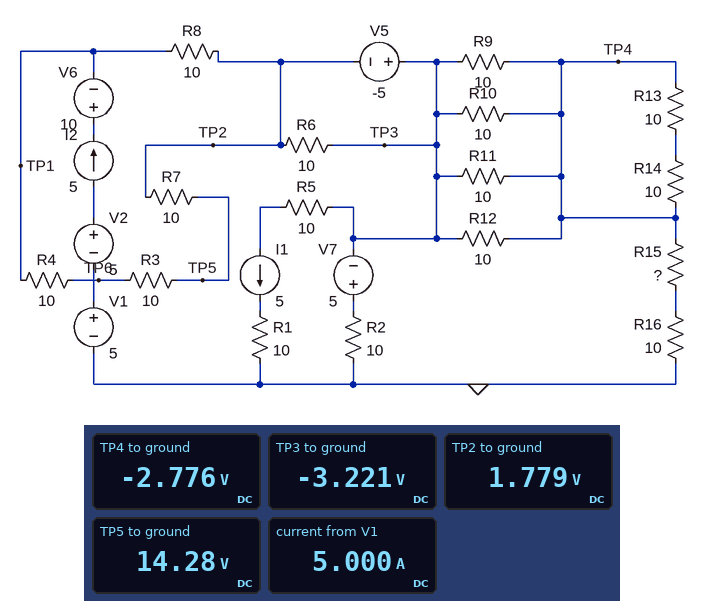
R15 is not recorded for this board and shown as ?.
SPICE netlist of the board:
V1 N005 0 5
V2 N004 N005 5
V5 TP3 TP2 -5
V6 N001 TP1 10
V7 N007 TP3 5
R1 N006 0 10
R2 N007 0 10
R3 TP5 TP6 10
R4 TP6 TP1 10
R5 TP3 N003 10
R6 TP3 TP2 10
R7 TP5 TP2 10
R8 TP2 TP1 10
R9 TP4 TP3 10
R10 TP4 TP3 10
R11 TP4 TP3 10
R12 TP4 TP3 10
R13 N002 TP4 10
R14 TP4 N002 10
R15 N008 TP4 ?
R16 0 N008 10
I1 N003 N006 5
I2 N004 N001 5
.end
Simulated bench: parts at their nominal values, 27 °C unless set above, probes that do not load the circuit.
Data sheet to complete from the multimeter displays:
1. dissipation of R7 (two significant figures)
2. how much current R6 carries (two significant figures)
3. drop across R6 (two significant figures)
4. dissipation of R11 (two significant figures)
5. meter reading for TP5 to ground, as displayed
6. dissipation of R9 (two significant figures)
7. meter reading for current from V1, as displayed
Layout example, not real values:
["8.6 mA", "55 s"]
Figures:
["16 W", "500 mA", "5.0 V", "20 mW", "14.28 V", "20 mW", "5.000 A"]
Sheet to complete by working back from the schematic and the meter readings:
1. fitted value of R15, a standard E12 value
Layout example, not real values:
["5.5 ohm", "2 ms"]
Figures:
["5.6 Ω"]
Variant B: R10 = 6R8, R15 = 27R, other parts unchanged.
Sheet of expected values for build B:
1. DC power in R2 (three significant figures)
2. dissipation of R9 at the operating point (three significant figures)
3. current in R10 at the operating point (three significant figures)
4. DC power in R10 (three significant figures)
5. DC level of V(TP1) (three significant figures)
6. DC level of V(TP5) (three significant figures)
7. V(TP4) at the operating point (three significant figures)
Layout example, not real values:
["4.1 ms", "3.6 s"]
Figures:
["103 mW", "5.16 mW", "33.4 mA", "7.59 mW", "38.5 V", "13.5 V", "-3.76 V"]
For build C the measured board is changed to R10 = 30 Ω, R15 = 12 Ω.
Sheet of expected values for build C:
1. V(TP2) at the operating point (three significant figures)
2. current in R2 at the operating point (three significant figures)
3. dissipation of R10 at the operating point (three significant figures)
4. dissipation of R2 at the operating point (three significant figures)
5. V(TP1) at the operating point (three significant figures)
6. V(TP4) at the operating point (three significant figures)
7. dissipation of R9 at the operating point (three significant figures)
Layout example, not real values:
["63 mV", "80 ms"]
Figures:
["1.43 V", "143 mA", "6.12 mW", "204 mW", "38.9 V", "-3.14 V", "18.4 mW"]
